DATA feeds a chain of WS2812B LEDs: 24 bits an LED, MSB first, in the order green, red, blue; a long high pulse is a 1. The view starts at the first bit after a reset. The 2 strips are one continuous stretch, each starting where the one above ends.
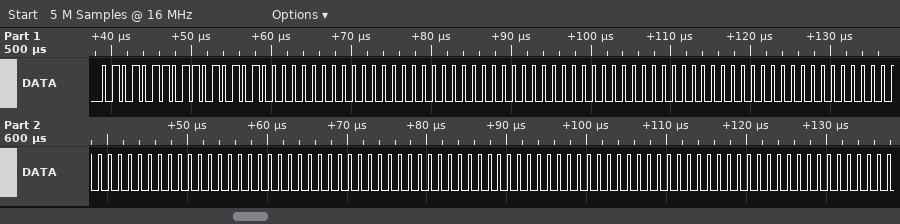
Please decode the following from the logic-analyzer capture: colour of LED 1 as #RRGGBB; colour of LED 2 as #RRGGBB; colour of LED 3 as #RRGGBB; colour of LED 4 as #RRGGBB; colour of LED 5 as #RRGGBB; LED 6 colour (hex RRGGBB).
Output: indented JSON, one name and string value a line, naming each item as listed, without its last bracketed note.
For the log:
{
  "colour of LED 1 as #RRGGBB": "#D55600",
  "colour of LED 2 as #RRGGBB": "#000000",
  "colour of LED 3 as #RRGGBB": "#000000",
  "colour of LED 4 as #RRGGBB": "#000000",
  "colour of LED 5 as #RRGGBB": "#000000",
  "LED 6 colour": "#000000"
}
